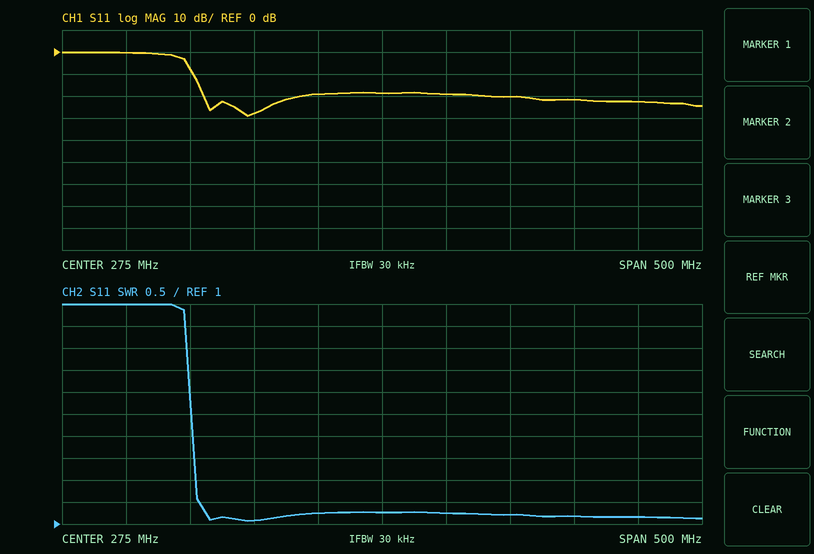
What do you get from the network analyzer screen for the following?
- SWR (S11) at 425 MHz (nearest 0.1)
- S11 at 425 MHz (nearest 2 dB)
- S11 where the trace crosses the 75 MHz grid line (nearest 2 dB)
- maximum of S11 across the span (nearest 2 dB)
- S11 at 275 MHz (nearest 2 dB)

1.2
-22 dB
0 dB
0 dB
-18 dB
